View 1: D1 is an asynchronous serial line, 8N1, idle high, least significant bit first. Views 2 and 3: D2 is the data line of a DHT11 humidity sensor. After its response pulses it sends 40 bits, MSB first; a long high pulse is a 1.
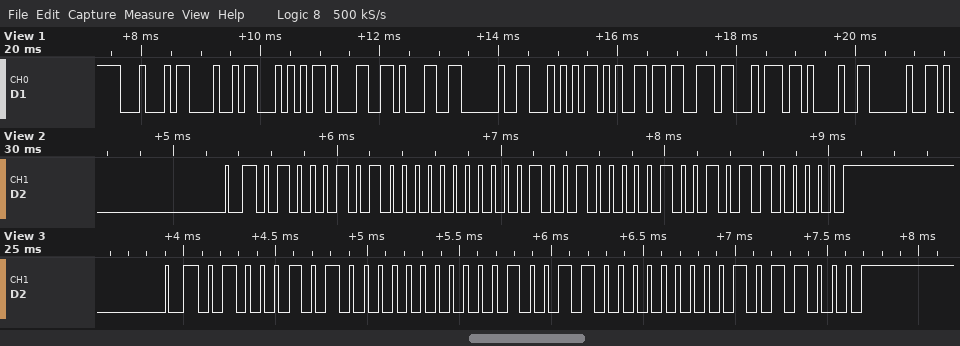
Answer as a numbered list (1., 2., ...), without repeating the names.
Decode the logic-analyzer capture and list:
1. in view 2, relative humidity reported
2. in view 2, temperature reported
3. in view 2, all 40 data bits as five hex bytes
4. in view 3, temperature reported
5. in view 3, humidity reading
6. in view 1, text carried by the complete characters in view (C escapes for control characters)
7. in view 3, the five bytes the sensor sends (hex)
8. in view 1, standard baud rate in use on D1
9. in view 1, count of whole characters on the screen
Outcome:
1. 69 %
2. 18.9 °C
3. 45 00 12 09 60
4. 19.0 °C
5. 69 %
6. "DHT11 Test! "
7. 45 00 13 00 58
8. 9600 baud
9. 12
